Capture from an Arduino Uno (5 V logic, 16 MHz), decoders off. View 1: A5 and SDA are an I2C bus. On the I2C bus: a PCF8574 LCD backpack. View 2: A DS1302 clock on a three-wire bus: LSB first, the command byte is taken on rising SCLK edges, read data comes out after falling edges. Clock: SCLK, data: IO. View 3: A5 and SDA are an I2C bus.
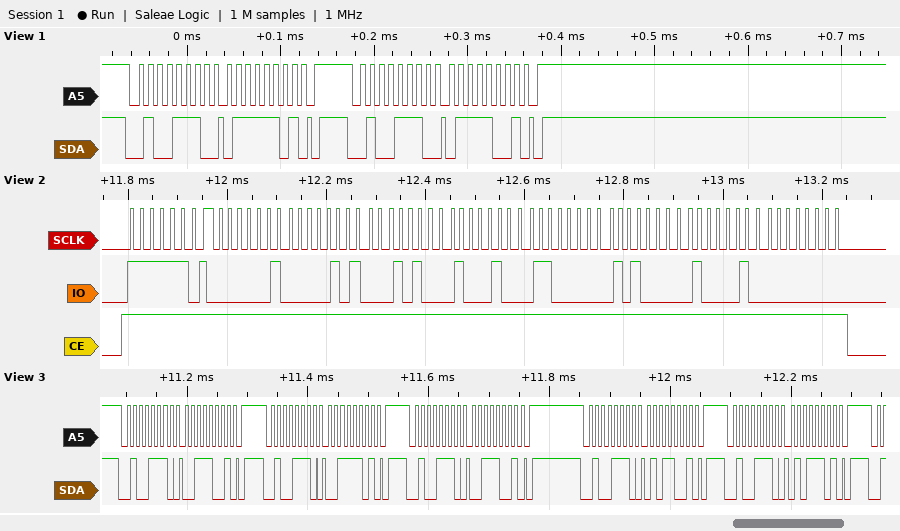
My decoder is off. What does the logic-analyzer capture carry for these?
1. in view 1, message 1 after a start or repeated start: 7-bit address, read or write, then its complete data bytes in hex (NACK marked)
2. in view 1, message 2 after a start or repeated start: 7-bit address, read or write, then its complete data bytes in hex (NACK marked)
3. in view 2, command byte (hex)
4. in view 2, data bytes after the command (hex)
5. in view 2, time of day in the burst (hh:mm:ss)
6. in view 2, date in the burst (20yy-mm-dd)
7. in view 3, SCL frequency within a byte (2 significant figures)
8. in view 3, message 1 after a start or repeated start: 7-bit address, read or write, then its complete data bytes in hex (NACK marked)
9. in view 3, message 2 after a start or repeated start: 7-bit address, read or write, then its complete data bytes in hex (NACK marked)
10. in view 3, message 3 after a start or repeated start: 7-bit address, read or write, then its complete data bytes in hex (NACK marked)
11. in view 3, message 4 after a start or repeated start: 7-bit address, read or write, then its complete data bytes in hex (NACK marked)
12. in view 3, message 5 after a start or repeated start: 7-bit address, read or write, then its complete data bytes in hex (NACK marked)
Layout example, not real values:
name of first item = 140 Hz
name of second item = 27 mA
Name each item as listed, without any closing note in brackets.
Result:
in view 1, message 1 after a start or repeated start: 7-bit address, read or write, then its complete data bytes in hex = 0x27 write: 7D
in view 1, message 2 after a start or repeated start: 7-bit address, read or write, then its complete data bytes in hex = 0x27 write: 79
in view 2, command byte = 0xBF
in view 2, data bytes after the command = 40 50 14 11 03 05 21 00
in view 2, time of day in the burst = 14:50:40
in view 2, date in the burst = 2021-03-11
in view 3, SCL frequency within a byte = 100 kHz
in view 3, message 1 after a start or repeated start: 7-bit address, read or write, then its complete data bytes in hex = 0x27 write: 39
in view 3, message 2 after a start or repeated start: 7-bit address, read or write, then its complete data bytes in hex = 0x27 write: 3D
in view 3, message 3 after a start or repeated start: 7-bit address, read or write, then its complete data bytes in hex = 0x27 write: 39
in view 3, message 4 after a start or repeated start: 7-bit address, read or write, then its complete data bytes in hex = 0x27 write: 59
in view 3, message 5 after a start or repeated start: 7-bit address, read or write, then its complete data bytes in hex = 0x27 write: 5D
